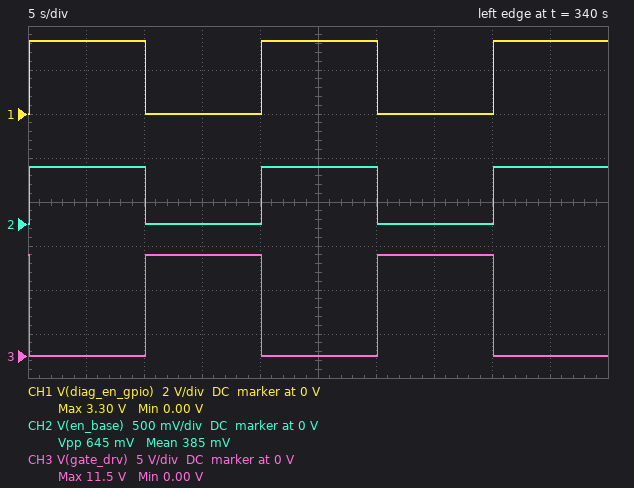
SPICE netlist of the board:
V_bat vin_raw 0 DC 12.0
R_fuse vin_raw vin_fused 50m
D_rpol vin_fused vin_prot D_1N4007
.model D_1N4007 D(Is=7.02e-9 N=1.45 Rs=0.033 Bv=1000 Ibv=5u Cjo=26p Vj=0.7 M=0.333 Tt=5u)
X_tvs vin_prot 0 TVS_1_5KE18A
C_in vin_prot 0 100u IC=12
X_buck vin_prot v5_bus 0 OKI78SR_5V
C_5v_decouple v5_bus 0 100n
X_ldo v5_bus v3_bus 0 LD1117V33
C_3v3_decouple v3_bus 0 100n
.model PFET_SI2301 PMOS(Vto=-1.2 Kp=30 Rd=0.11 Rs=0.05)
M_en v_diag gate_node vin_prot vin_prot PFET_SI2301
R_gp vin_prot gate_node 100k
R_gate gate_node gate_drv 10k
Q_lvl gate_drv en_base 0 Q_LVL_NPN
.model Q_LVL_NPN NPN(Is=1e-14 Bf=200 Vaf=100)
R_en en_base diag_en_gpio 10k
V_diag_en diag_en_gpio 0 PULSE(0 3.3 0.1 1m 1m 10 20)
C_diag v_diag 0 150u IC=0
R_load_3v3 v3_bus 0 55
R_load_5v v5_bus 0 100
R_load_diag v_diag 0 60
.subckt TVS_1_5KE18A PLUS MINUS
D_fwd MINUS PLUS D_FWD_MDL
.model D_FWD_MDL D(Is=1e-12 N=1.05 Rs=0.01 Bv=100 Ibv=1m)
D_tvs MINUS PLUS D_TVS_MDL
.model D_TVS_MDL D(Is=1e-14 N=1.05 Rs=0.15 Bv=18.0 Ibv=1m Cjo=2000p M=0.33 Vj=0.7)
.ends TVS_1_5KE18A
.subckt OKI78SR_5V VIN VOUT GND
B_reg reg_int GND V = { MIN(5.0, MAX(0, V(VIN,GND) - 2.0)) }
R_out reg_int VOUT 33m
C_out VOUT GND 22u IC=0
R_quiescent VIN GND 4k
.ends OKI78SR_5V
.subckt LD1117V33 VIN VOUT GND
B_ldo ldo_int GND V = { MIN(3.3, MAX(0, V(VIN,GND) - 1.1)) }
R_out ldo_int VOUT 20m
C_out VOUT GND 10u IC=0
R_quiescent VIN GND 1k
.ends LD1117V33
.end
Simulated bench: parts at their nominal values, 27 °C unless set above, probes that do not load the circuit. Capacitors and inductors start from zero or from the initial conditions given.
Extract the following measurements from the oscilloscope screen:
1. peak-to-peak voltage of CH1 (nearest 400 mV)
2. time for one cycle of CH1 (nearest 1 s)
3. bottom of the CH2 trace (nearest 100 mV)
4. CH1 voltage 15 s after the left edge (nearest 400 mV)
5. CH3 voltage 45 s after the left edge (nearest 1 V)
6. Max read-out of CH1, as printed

3.2 V
20 s
0 V
0 V
0 V
3.30 V
